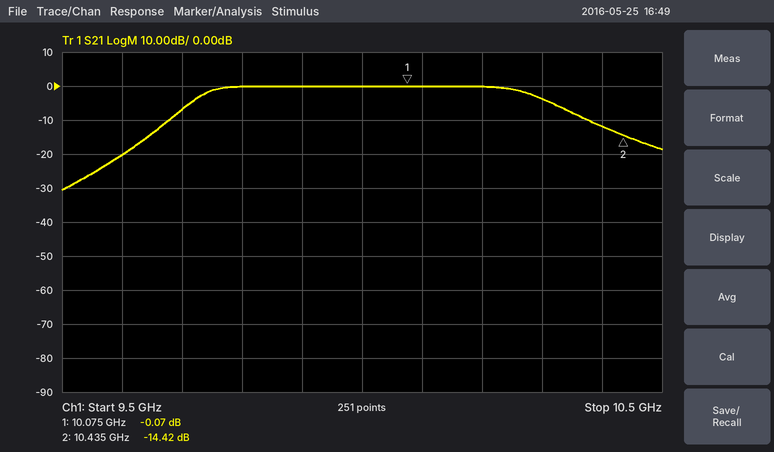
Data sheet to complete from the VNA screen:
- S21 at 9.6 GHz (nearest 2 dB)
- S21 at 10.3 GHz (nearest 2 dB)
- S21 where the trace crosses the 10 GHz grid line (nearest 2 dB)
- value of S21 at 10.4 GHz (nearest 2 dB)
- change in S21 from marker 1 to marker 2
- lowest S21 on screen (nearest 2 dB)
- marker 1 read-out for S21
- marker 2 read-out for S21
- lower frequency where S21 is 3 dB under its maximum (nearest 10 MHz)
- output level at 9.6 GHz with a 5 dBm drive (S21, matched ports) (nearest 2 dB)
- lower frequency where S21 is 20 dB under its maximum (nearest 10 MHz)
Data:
-20 dB
-4 dB
0 dB
-12 dB
-14.35 dB
-30 dB
-0.07 dB
-14.42 dB
9.73 GHz
-16 dBm
9.60 GHz
